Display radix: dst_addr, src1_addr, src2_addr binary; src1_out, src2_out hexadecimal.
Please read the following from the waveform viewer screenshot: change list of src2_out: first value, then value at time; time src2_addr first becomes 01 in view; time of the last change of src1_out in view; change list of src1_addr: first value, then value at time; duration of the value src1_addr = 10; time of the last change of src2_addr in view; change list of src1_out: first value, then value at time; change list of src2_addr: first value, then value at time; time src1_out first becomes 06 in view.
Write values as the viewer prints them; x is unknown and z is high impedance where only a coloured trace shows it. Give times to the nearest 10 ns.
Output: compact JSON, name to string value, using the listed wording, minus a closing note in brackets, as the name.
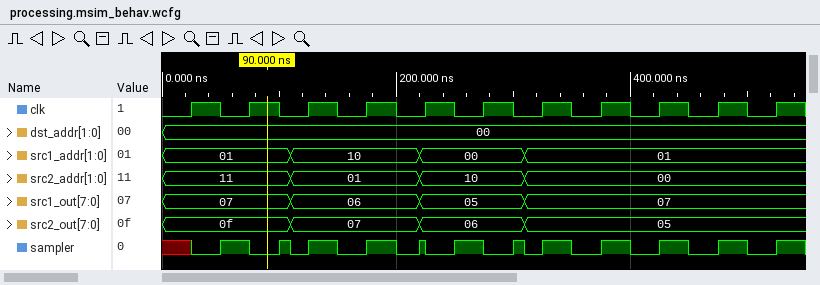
{"change list of src2_out: first value, then value at time": "0f, 07 at 110 ns, 06 at 220 ns, 05 at 310 ns", "time src2_addr first becomes 01 in view": "110 ns", "time of the last change of src1_out in view": "310 ns", "change list of src1_addr: first value, then value at time": "01, 10 at 110 ns, 00 at 220 ns, 01 at 310 ns", "duration of the value src1_addr = 10": "110 ns", "time of the last change of src2_addr in view": "310 ns", "change list of src1_out: first value, then value at time": "07, 06 at 110 ns, 05 at 220 ns, 07 at 310 ns", "change list of src2_addr: first value, then value at time": "11, 01 at 110 ns, 10 at 220 ns, 00 at 310 ns", "time src1_out first becomes 06 in view": "110 ns"}
